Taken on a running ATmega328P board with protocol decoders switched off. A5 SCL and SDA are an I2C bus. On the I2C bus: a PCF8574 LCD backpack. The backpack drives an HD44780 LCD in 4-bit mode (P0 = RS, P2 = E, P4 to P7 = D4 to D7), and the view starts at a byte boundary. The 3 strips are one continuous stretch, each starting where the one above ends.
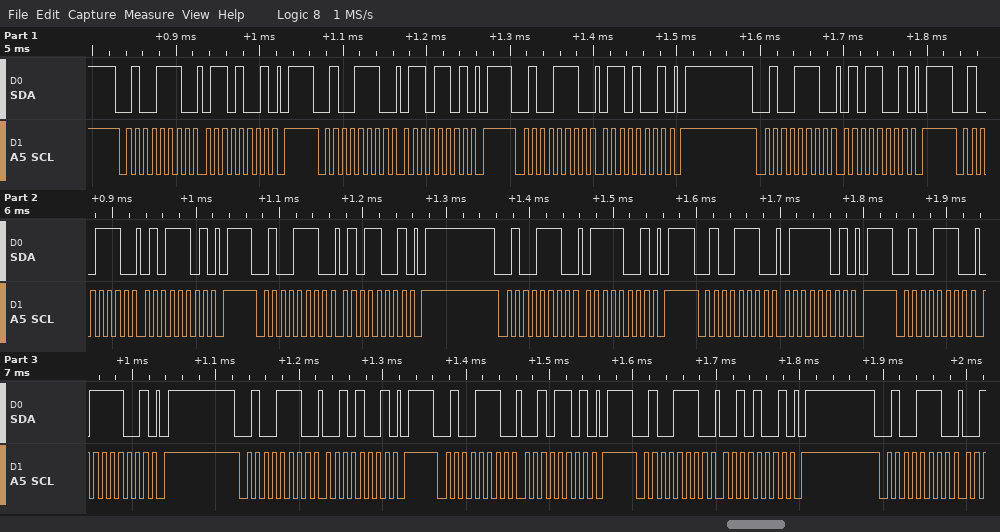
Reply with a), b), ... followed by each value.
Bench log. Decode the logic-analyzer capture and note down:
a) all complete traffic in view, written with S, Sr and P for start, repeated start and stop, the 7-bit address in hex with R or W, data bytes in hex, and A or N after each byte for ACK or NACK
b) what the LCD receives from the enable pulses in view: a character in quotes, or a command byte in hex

a) S 27W A 69 A P S 27W A 6D A P S 27W A 69 A P S 27W A 59 A P S 27W A 5D A P S 27W A 59 A P S 27W A 79 A P S 27W A 7D A P S 27W A 79 A P S 27W A 29 A P S 27W A 2D A P S 27W A 29 A P S 27W A
b) 'e' 'r'
